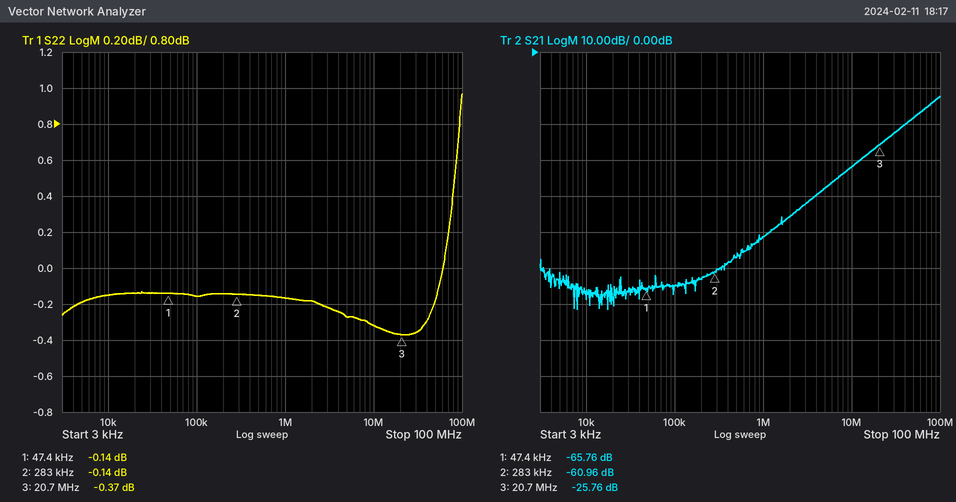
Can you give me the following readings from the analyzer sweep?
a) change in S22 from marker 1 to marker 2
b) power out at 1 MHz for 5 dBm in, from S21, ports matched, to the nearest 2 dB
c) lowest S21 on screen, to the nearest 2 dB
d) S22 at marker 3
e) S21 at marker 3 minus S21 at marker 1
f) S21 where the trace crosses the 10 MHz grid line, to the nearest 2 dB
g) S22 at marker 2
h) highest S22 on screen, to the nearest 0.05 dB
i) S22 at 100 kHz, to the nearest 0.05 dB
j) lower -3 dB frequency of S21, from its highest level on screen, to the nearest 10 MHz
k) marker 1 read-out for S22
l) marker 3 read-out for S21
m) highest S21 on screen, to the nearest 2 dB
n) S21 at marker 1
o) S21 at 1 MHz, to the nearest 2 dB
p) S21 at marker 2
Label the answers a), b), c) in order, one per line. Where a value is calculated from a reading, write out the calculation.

a) -0.14 − (-0.14) = 0.00 dB
b) 5 dBm + (-52 dB) = -46 dBm
c) -72 dB
d) -0.37 dB
e) -25.76 − (-65.76) = 40.00 dB
f) -32 dB
g) -0.14 dB
h) 0.95 dB
i) -0.15 dB
j) 70 MHz
k) -0.14 dB
l) -25.76 dB
m) -12 dB
n) -65.76 dB
o) -52 dB
p) -60.96 dB
